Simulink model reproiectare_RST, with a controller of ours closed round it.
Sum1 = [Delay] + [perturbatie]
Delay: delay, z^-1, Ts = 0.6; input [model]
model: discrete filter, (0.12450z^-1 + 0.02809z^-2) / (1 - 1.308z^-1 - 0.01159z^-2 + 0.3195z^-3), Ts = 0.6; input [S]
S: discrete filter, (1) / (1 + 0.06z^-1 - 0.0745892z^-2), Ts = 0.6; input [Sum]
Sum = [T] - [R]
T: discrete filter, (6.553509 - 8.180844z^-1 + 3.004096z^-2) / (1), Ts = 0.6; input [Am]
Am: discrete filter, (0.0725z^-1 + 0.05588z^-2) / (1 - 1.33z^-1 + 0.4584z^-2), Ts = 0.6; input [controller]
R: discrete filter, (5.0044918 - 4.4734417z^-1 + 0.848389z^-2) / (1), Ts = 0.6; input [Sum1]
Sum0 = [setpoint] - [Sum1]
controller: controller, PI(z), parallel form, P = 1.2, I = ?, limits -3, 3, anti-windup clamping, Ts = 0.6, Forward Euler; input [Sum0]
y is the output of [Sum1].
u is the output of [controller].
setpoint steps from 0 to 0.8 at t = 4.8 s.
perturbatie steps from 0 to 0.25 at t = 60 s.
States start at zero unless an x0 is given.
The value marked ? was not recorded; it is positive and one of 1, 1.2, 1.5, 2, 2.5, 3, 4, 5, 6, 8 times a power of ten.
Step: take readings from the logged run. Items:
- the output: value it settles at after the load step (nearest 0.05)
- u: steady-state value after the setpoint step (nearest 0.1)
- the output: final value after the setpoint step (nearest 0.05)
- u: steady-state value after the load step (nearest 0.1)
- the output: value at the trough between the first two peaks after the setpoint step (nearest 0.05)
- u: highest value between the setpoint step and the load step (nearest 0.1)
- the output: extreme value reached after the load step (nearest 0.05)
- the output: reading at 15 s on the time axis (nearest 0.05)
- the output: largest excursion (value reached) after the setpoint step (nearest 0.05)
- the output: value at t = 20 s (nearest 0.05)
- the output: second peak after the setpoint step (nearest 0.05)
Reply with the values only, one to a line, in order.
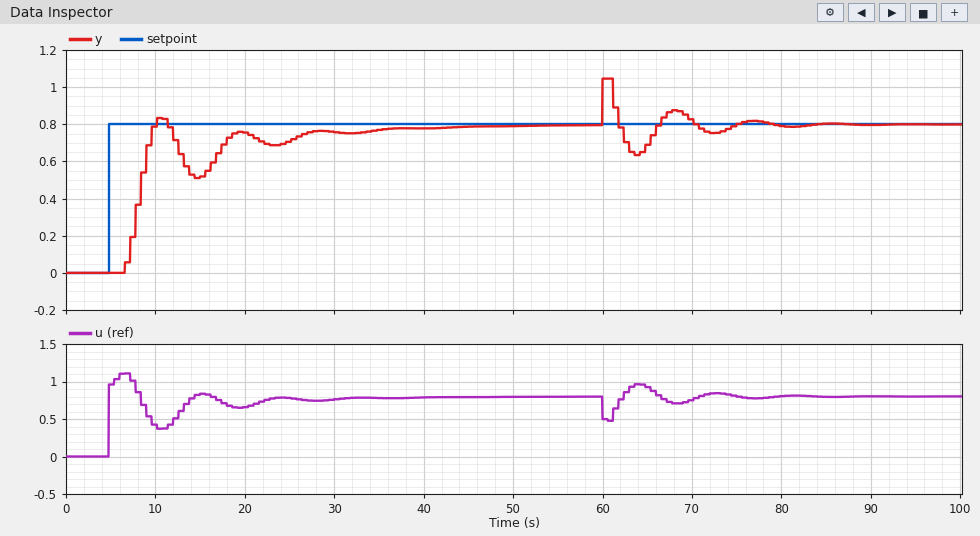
0.80
0.8
0.80
0.8
0.50
1.1
1.05
0.50
0.85
0.75
0.75
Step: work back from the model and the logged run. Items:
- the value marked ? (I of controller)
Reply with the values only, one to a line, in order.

0.15
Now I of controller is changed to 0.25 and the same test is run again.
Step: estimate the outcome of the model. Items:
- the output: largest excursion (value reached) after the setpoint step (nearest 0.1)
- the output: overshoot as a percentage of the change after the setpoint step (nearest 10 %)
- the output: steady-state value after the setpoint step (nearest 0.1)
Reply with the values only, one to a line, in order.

1.0
20 %
0.8
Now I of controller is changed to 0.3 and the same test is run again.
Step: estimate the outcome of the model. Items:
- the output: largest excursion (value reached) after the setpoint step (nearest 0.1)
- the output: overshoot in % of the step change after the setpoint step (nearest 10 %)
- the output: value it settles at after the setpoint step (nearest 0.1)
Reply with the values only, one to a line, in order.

1.0
30 %
0.8
